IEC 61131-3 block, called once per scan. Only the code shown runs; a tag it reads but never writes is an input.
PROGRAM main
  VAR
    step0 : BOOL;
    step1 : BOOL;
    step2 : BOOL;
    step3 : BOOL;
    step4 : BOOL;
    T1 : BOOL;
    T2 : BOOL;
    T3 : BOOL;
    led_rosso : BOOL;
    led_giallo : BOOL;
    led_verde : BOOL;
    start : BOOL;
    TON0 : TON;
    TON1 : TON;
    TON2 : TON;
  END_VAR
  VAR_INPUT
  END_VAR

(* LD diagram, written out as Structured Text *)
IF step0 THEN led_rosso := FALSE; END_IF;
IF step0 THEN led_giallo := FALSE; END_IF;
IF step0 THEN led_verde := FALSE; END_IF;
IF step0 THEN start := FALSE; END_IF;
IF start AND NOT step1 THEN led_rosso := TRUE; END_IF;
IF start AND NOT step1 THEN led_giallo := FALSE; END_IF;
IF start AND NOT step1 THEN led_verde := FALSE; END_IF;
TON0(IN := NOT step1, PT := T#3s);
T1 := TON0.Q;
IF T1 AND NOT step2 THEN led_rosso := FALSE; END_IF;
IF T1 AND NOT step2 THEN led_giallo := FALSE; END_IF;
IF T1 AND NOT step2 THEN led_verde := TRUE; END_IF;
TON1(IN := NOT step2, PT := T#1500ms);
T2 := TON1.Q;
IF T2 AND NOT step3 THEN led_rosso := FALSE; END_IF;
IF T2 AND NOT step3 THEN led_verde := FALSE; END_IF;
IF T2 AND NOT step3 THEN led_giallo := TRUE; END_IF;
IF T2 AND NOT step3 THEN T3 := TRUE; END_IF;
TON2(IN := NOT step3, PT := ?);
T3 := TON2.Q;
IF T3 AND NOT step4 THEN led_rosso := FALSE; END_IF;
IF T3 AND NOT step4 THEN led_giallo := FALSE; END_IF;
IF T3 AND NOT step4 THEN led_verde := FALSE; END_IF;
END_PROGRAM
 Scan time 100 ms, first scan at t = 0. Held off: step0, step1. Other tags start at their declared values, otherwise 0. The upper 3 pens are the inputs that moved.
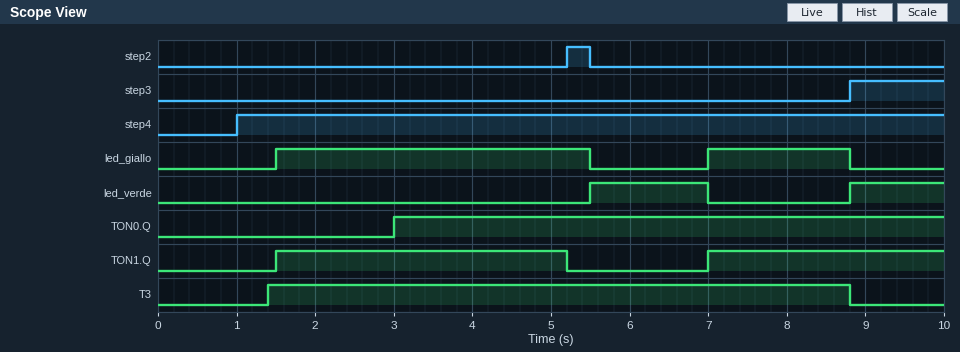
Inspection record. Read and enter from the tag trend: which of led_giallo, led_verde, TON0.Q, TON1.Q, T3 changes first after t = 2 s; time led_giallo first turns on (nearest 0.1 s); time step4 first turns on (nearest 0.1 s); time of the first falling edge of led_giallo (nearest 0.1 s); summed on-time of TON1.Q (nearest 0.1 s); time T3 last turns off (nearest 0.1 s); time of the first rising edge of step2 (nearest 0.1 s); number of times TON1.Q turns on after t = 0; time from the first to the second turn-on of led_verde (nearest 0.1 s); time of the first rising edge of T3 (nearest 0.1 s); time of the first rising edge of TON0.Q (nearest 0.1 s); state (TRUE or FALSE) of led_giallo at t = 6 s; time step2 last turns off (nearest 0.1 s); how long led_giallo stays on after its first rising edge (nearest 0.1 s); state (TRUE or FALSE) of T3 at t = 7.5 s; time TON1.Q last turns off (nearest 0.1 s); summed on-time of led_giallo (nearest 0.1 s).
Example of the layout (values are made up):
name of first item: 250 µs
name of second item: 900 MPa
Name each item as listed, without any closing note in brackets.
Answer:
which of led_giallo, led_verde, TON0.Q, TON1.Q, T3 changes first after t = 2 s: TON0.Q
time led_giallo first turns on: 1.5 s
time step4 first turns on: 1.0 s
time of the first falling edge of led_giallo: 5.5 s
summed on-time of TON1.Q: 6.7 s
time T3 last turns off: 8.8 s
time of the first rising edge of step2: 5.2 s
number of times TON1.Q turns on after t = 0: 2
time from the first to the second turn-on of led_verde: 3.3 s
time of the first rising edge of T3: 1.4 s
time of the first rising edge of TON0.Q: 3.0 s
state (TRUE or FALSE) of led_giallo at t = 6 s: FALSE
time step2 last turns off: 5.5 s
how long led_giallo stays on after its first rising edge: 4.0 s
state (TRUE or FALSE) of T3 at t = 7.5 s: TRUE
time TON1.Q last turns off: 5.2 s
summed on-time of led_giallo: 5.8 s
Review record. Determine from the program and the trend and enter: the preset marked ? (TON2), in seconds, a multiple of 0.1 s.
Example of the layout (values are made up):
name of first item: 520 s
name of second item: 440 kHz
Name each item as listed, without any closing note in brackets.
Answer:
the preset marked ? (TON2), in seconds, a multiple of 0.1 s: 1.4 s
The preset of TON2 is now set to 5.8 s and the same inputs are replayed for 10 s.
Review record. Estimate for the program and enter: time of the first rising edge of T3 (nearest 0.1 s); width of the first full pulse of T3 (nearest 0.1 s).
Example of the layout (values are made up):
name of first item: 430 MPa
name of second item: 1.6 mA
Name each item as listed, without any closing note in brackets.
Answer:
time of the first rising edge of T3: 5.8 s
width of the first full pulse of T3: 3.0 s
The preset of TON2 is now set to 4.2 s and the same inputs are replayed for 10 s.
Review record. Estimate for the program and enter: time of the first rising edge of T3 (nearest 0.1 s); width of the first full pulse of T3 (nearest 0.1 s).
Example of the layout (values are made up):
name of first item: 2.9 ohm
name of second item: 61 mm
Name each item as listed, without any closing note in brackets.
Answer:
time of the first rising edge of T3: 4.2 s
width of the first full pulse of T3: 4.6 s
